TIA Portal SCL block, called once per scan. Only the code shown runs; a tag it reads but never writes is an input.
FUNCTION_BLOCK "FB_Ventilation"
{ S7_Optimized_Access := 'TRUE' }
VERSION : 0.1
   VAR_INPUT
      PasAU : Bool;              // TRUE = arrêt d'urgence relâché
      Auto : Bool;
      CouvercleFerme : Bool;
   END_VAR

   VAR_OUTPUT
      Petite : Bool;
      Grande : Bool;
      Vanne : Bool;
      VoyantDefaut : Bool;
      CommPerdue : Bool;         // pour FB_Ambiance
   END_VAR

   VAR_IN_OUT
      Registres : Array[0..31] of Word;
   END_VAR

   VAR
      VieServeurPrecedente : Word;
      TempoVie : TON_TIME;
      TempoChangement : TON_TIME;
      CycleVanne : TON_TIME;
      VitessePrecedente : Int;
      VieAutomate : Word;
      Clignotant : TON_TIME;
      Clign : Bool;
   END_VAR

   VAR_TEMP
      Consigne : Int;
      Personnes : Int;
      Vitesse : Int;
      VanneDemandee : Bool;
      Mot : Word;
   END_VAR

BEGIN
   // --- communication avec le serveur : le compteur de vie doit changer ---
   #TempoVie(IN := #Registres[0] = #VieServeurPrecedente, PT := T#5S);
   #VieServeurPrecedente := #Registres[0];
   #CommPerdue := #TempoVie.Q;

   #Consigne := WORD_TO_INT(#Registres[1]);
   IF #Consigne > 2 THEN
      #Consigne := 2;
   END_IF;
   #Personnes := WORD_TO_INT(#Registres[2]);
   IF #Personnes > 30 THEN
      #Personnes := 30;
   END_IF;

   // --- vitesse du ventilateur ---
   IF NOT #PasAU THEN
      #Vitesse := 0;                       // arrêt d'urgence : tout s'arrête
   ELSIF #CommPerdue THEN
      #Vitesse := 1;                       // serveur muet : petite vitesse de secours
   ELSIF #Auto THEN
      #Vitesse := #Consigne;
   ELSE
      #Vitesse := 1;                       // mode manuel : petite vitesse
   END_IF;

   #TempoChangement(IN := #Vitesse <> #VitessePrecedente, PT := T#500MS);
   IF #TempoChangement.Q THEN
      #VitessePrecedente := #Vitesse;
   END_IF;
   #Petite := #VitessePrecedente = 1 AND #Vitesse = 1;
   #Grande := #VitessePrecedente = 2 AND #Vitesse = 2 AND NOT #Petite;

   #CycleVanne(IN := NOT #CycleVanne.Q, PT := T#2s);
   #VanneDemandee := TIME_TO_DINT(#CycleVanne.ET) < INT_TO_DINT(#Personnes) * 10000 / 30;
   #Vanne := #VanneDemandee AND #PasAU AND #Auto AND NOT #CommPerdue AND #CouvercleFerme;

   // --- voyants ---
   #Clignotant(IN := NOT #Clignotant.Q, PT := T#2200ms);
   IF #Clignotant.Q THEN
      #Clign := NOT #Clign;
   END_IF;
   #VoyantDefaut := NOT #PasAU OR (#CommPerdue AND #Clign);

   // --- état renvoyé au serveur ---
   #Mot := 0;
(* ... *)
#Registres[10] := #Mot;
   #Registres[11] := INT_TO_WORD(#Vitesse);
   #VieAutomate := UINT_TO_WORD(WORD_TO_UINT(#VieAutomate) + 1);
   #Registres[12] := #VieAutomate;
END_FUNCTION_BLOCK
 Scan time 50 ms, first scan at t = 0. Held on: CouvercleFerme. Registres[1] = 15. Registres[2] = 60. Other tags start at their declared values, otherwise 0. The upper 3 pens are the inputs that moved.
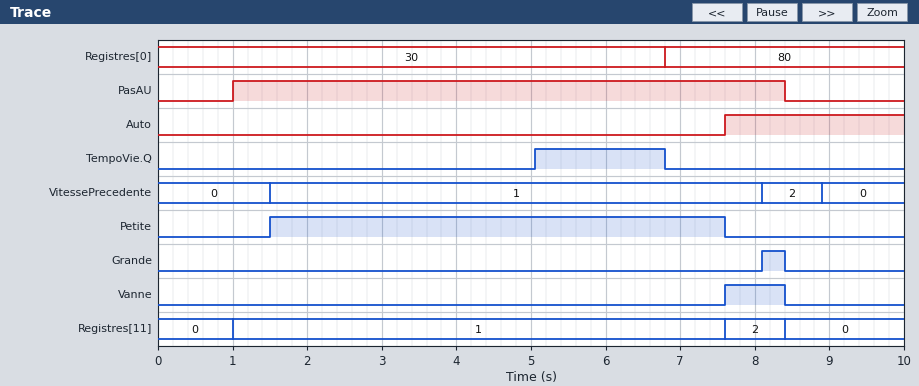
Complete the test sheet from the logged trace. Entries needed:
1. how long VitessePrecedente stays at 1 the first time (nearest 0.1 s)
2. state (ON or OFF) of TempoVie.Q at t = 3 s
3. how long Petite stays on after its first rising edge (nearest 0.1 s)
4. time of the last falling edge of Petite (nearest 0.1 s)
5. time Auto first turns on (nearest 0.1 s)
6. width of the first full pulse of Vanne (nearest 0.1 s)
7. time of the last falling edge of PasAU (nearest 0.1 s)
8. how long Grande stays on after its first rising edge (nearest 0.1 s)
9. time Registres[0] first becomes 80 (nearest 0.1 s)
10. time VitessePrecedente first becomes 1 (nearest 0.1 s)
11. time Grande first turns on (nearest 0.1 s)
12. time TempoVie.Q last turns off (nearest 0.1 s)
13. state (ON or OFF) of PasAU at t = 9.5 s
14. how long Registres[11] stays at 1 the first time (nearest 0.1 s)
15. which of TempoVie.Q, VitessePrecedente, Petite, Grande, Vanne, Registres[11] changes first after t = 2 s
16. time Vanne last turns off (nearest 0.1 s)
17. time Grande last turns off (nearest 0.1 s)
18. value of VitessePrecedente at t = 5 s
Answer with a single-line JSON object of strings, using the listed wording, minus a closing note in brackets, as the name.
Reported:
{"how long VitessePrecedente stays at 1 the first time": "6.6 s", "state (ON or OFF) of TempoVie.Q at t = 3 s": "OFF", "how long Petite stays on after its first rising edge": "6.1 s", "time of the last falling edge of Petite": "7.6 s", "time Auto first turns on": "7.6 s", "width of the first full pulse of Vanne": "0.8 s", "time of the last falling edge of PasAU": "8.4 s", "how long Grande stays on after its first rising edge": "0.3 s", "time Registres[0] first becomes 80": "6.8 s", "time VitessePrecedente first becomes 1": "1.5 s", "time Grande first turns on": "8.1 s", "time TempoVie.Q last turns off": "6.8 s", "state (ON or OFF) of PasAU at t = 9.5 s": "OFF", "how long Registres[11] stays at 1 the first time": "6.6 s", "which of TempoVie.Q, VitessePrecedente, Petite, Grande, Vanne, Registres[11] changes first after t = 2 s": "TempoVie.Q", "time Vanne last turns off": "8.4 s", "time Grande last turns off": "8.4 s", "value of VitessePrecedente at t = 5 s": "1"}
